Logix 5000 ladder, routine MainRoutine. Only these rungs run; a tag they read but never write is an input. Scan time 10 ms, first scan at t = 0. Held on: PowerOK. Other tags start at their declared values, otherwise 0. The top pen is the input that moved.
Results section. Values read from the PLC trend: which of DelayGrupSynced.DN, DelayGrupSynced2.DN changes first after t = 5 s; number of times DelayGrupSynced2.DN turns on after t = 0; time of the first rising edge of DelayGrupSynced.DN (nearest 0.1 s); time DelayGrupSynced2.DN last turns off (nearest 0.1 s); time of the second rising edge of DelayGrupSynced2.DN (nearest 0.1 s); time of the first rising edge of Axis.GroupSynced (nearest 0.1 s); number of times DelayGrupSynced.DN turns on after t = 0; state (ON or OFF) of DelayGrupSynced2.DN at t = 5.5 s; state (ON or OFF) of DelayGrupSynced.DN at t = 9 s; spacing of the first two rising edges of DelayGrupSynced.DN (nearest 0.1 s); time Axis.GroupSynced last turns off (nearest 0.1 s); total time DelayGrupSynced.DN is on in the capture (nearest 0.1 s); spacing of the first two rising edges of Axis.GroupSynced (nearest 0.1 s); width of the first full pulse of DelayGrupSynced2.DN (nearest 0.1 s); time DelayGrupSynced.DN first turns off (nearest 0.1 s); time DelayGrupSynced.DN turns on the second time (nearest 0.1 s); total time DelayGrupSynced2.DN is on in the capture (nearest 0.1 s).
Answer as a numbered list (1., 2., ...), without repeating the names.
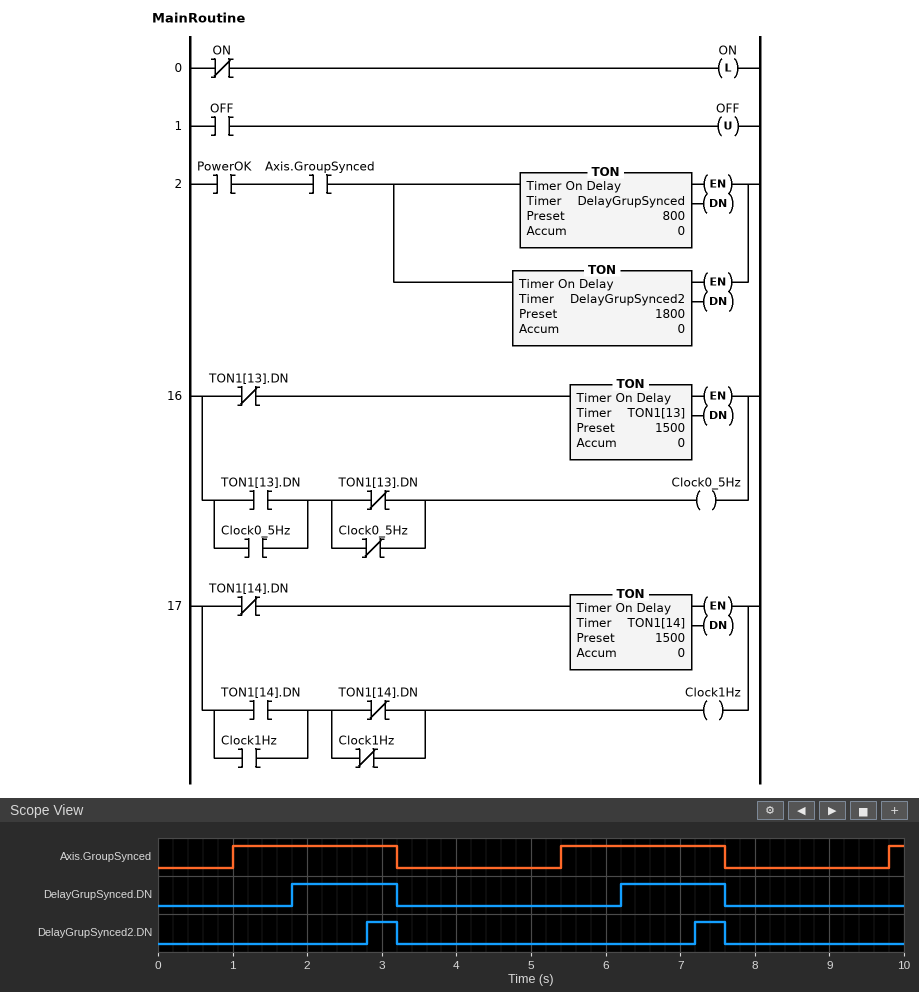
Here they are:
1. DelayGrupSynced.DN
2. 2
3. 1.8 s
4. 7.6 s
5. 7.2 s
6. 1.0 s
7. 2
8. OFF
9. OFF
10. 4.4 s
11. 7.6 s
12. 2.8 s
13. 4.4 s
14. 0.4 s
15. 3.2 s
16. 6.2 s
17. 0.8 s
